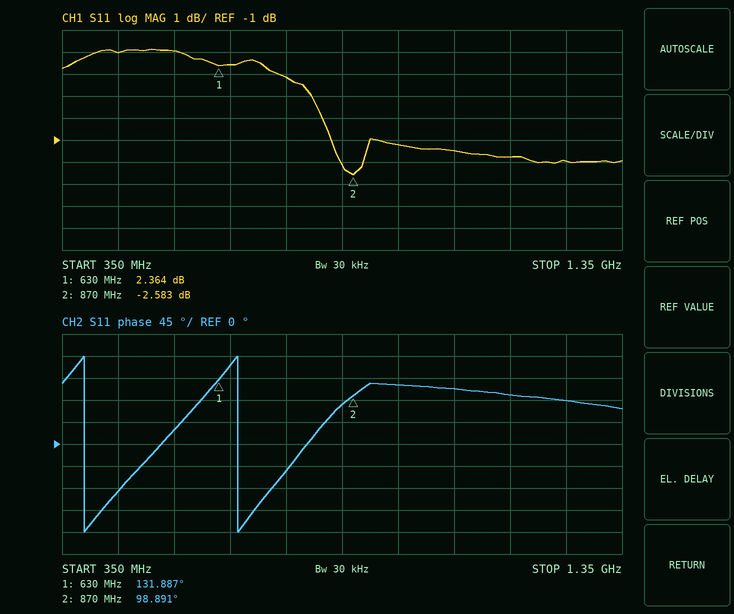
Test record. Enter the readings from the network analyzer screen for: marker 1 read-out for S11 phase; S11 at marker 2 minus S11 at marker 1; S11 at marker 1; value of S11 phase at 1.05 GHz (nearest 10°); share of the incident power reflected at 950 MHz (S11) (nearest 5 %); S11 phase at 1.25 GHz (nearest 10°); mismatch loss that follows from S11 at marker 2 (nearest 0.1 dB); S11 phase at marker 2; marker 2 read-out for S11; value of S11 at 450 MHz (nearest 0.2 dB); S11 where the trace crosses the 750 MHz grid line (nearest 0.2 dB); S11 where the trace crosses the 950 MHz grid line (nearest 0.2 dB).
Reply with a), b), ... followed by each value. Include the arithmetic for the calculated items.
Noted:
a) 131.887°
b) -2.583 − (2.364) = -4.947 dB
c) 2.364 dB
d) 110°
e) 10^(-1.2/10) ≈ 75.9 %, so 75 % to the nearest 5 %
f) 90°
g) −10 log10(1 − 10^(-2.583/10)) ≈ 3.5 dB
h) 98.891°
i) -2.583 dB
j) 3.0 dB
k) 1.8 dB
l) -1.2 dB
